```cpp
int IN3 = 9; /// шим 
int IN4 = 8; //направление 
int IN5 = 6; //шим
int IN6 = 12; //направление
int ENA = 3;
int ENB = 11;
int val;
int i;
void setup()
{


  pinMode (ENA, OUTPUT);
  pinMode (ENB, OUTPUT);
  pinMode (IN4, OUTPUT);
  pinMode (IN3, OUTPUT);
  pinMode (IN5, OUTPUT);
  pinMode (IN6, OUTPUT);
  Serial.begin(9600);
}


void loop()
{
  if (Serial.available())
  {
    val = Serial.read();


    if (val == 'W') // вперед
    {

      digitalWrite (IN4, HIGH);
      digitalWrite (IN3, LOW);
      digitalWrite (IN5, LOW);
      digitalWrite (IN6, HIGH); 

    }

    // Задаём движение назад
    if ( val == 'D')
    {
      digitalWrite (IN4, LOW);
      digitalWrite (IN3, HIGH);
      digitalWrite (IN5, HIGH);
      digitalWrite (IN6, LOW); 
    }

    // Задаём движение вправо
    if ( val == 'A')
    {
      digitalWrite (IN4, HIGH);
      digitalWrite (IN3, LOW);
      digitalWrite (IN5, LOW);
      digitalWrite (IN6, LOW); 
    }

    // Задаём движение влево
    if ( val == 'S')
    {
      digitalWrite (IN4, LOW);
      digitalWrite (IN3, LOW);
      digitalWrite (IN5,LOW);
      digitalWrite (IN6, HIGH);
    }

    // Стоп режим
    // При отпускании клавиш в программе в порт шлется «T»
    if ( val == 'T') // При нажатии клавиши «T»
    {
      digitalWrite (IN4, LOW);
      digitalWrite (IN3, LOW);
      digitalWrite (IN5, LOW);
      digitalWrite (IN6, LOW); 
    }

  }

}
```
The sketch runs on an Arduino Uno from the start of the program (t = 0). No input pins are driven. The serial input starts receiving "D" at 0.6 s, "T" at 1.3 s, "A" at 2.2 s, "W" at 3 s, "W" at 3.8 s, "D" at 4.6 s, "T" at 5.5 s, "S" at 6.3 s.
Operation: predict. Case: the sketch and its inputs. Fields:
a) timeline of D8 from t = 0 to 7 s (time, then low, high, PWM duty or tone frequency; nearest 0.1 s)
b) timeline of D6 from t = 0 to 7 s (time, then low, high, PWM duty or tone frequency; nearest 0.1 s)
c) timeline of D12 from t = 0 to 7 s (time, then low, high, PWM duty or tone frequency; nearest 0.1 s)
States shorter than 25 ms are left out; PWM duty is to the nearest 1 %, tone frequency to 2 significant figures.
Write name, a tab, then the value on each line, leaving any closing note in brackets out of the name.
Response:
timeline of D8 from t = 0 to 7 s	0 s low; 2.2 s high; 4.6 s low
timeline of D6 from t = 0 to 7 s	0 s low; 0.6 s high; 1.3 s low; 4.6 s high; 5.5 s low
timeline of D12 from t = 0 to 7 s	0 s low; 3 s high; 4.6 s low; 6.3 s high
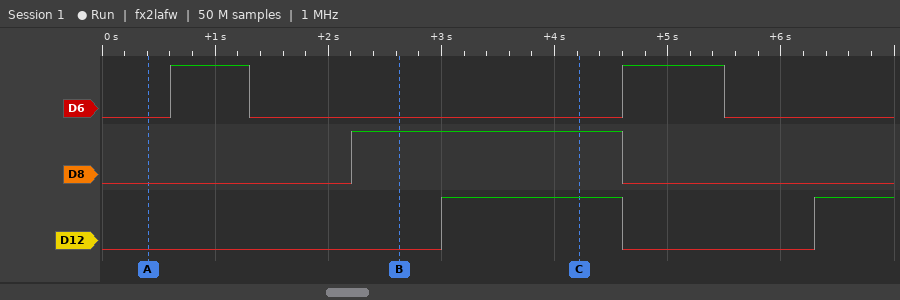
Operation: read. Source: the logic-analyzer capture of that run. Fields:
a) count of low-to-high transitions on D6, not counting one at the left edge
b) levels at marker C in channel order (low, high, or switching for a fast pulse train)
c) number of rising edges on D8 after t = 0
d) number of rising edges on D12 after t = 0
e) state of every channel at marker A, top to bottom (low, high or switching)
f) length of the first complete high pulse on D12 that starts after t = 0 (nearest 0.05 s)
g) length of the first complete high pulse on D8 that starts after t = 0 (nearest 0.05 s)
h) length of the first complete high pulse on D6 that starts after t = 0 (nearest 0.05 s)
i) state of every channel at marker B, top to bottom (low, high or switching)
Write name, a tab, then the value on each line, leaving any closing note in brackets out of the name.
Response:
count of low-to-high transitions on D6, not counting one at the left edge	2
levels at marker C in channel order	D6 low, D8 high, D12 high
number of rising edges on D8 after t = 0	1
number of rising edges on D12 after t = 0	2
state of every channel at marker A, top to bottom	D6 low, D8 low, D12 low
length of the first complete high pulse on D12 that starts after t = 0	1.60 s
length of the first complete high pulse on D8 that starts after t = 0	2.40 s
length of the first complete high pulse on D6 that starts after t = 0	0.70 s
state of every channel at marker B, top to bottom	D6 low, D8 high, D12 low
